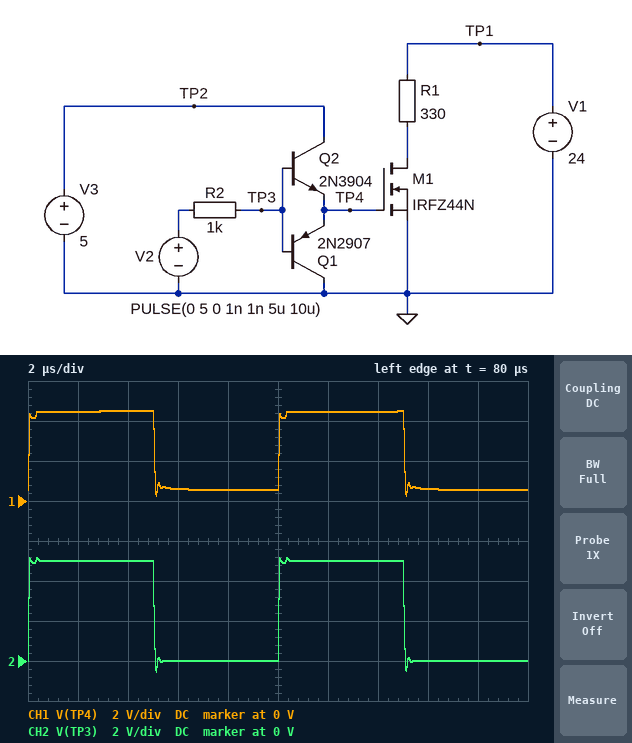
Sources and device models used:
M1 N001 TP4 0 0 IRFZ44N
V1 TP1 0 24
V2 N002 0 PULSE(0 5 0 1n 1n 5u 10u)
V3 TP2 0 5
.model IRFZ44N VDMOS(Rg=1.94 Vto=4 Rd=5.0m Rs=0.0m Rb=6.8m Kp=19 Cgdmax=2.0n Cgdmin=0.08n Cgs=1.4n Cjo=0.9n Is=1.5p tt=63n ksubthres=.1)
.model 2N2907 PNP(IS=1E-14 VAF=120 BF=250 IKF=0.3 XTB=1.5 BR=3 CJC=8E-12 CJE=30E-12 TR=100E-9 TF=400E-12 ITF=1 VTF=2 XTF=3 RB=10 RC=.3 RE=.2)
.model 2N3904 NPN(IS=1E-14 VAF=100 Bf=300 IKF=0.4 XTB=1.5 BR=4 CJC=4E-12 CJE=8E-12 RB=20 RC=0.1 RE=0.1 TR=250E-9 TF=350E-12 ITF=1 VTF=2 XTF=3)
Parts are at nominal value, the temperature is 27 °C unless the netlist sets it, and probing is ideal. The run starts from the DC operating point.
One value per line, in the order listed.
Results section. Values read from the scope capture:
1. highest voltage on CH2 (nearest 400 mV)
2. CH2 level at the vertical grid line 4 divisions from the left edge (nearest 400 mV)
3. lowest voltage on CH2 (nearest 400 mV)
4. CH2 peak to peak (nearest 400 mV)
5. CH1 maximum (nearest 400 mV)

5.2 V
0 V
-400 mV
5.6 V
4.4 V
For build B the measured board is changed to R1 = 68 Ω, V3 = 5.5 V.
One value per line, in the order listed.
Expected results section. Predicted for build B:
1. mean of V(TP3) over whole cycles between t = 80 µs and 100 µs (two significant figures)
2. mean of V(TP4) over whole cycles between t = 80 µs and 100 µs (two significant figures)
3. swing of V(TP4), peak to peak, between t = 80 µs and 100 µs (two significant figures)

2.5 V
2.3 V
4.4 V
